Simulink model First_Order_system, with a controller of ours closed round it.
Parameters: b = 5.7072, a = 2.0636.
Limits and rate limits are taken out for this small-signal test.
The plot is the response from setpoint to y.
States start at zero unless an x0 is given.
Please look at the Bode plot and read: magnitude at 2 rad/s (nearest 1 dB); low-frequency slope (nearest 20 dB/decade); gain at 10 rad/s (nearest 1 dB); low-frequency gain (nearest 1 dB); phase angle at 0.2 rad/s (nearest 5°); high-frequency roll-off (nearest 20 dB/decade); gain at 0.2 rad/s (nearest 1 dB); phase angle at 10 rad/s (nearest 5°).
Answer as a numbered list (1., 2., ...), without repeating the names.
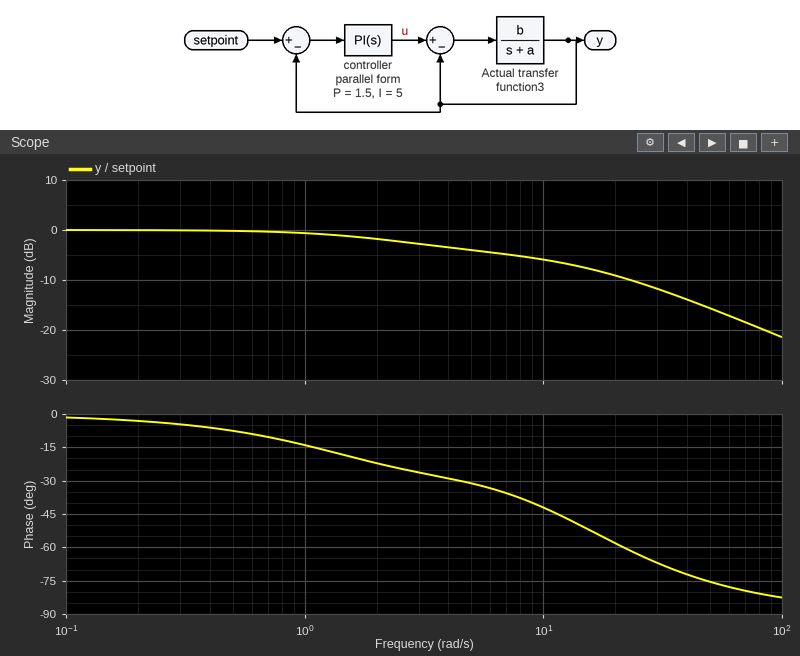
1. -2 dB
2. 0 dB/decade
3. -6 dB
4. 0 dB
5. -5°
6. -20 dB/decade
7. 0 dB
8. -40°
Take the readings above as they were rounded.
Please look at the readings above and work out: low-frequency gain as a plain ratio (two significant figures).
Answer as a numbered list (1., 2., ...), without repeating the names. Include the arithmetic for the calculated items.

1. 10^(0 / 20) = 1.0
